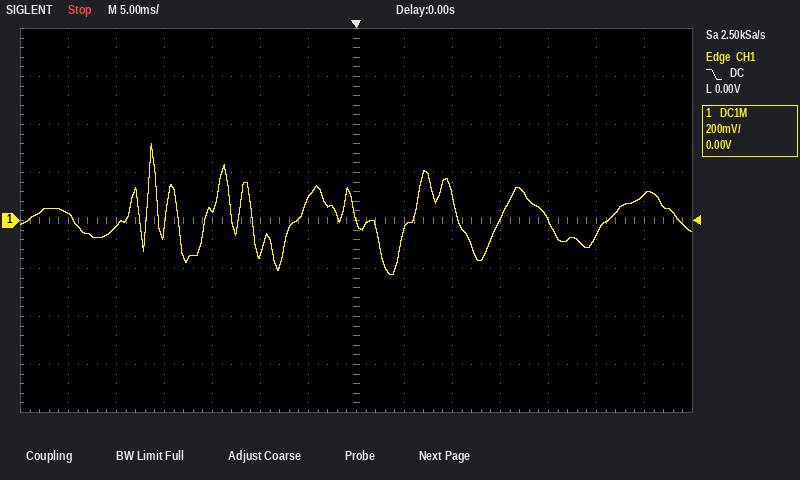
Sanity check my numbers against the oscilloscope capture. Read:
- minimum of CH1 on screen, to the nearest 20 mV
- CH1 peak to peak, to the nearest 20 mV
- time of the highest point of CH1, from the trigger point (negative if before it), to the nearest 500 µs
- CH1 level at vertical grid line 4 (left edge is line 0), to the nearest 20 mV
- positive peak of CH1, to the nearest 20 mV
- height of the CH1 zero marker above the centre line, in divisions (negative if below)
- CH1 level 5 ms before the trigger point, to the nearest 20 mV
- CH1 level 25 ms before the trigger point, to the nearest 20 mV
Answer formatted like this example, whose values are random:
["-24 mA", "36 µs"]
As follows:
["-220 mV", "540 mV", "-21.5 ms", "40 mV", "320 mV", "0.0 div", "100 mV", "-20 mV"]
